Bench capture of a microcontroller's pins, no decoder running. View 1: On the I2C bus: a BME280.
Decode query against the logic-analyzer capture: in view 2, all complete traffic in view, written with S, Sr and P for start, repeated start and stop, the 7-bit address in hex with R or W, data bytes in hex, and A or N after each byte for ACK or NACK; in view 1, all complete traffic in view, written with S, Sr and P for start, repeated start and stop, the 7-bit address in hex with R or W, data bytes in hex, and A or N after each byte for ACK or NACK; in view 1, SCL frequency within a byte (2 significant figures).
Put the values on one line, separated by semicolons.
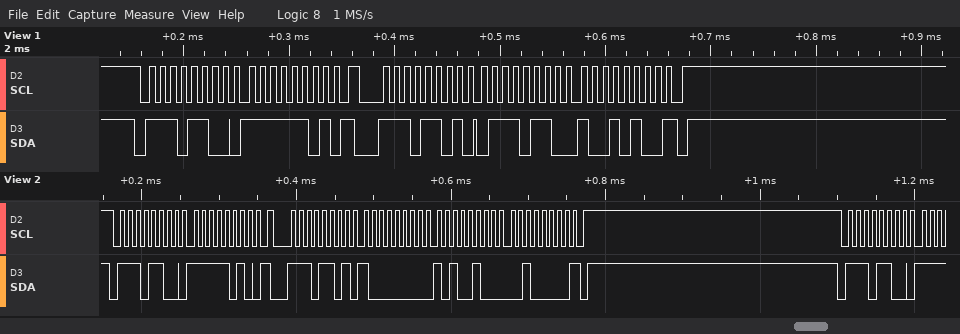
S 76W A FA A Sr 76R A 80 A A4 A 20 N P S 76W A; S 76W A FD A Sr 76R A 76 A 94 N P; 100 kHz
